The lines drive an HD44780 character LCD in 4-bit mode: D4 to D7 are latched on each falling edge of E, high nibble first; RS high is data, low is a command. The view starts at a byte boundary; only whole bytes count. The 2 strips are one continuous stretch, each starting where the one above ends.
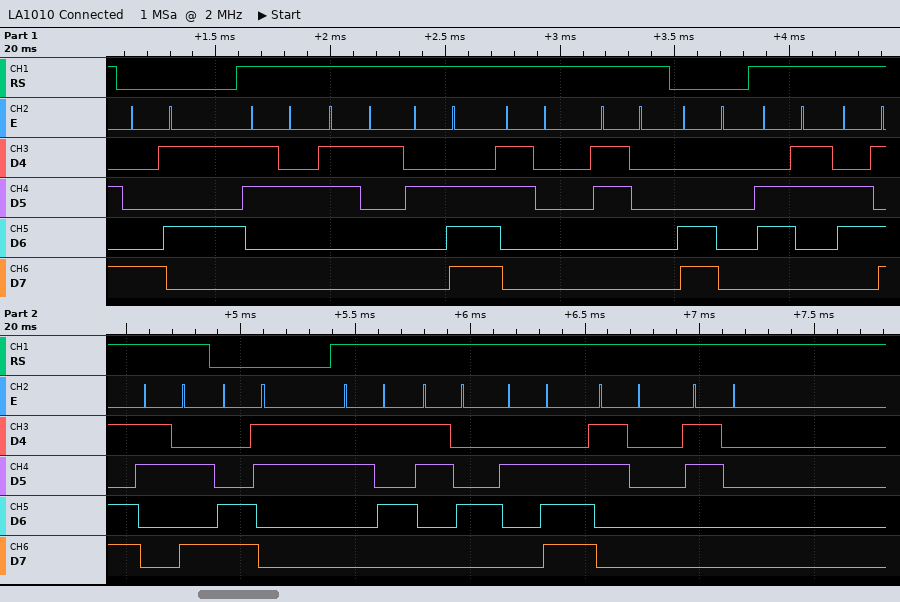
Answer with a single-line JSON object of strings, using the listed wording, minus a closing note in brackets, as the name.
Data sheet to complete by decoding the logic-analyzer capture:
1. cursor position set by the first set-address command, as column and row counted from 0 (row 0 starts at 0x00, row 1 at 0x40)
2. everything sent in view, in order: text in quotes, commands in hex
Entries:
{"cursor position set by the first set-address command, as column and row counted from 0": "column 5, row 0", "everything sent in view, in order: text in quotes, commands in hex": "0x85 \"21.00\" 0xC0 \"cm:\" 0xC3 \"54.00\""}
